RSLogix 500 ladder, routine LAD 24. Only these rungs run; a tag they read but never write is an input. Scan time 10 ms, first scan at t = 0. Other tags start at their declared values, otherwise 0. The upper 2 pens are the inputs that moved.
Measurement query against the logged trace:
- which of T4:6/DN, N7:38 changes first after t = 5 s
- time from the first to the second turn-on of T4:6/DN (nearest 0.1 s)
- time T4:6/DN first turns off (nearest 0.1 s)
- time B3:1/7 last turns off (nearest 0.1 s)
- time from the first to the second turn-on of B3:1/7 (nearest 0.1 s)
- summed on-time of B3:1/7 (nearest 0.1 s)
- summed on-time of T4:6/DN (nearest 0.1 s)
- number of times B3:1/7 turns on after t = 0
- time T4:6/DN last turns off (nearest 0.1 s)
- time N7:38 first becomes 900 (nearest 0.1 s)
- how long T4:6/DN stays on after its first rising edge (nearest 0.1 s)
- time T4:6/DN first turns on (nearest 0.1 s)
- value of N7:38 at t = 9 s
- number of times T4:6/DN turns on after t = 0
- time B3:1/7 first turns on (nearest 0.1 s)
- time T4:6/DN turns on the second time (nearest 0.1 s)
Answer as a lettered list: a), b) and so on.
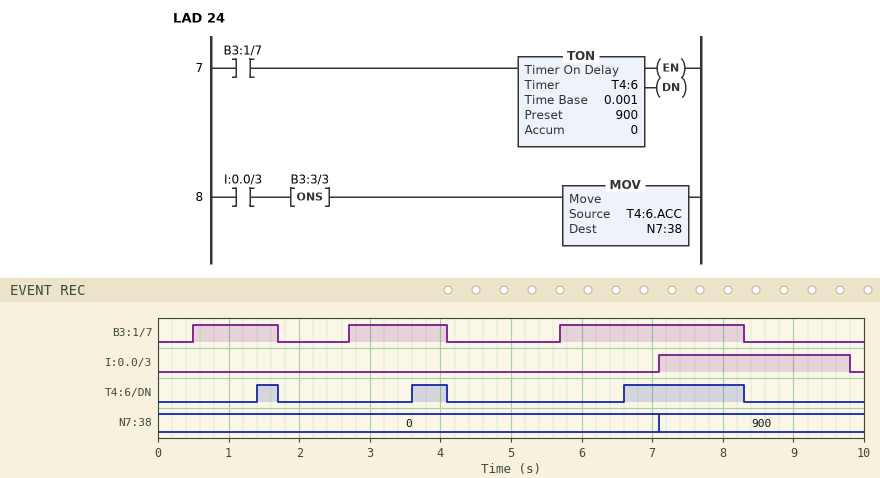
a) T4:6/DN
b) 2.2 s
c) 1.7 s
d) 8.3 s
e) 2.2 s
f) 5.2 s
g) 2.5 s
h) 3
i) 8.3 s
j) 7.1 s
k) 0.3 s
l) 1.4 s
m) 900
n) 3
o) 0.5 s
p) 3.6 s
